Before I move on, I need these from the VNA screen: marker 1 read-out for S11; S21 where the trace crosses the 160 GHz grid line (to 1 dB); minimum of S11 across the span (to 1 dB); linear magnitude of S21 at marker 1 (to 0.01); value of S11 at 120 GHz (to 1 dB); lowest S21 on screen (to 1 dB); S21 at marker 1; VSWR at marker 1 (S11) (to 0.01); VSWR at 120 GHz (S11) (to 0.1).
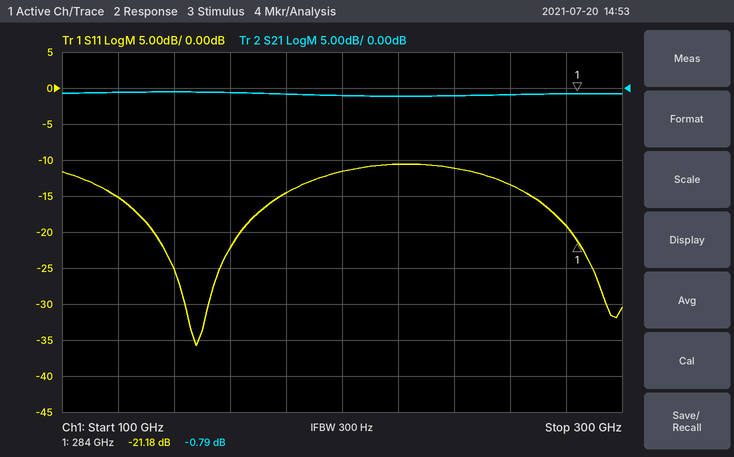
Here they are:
-21.18 dB
-1 dB
-36 dB
0.91
-15 dB
-1 dB
-0.79 dB
1.19
1.4
